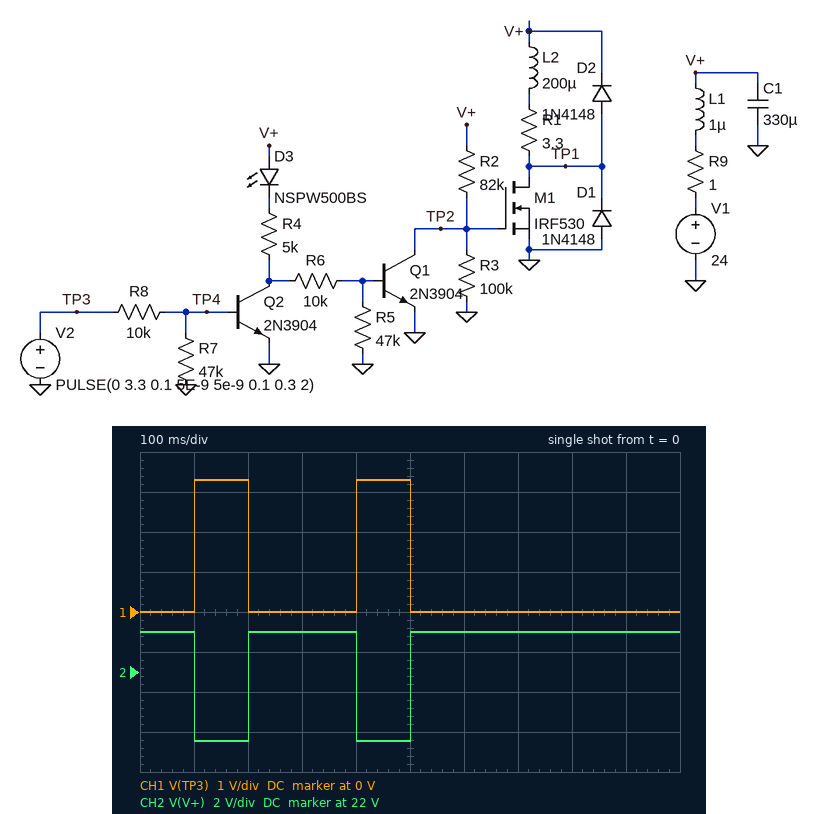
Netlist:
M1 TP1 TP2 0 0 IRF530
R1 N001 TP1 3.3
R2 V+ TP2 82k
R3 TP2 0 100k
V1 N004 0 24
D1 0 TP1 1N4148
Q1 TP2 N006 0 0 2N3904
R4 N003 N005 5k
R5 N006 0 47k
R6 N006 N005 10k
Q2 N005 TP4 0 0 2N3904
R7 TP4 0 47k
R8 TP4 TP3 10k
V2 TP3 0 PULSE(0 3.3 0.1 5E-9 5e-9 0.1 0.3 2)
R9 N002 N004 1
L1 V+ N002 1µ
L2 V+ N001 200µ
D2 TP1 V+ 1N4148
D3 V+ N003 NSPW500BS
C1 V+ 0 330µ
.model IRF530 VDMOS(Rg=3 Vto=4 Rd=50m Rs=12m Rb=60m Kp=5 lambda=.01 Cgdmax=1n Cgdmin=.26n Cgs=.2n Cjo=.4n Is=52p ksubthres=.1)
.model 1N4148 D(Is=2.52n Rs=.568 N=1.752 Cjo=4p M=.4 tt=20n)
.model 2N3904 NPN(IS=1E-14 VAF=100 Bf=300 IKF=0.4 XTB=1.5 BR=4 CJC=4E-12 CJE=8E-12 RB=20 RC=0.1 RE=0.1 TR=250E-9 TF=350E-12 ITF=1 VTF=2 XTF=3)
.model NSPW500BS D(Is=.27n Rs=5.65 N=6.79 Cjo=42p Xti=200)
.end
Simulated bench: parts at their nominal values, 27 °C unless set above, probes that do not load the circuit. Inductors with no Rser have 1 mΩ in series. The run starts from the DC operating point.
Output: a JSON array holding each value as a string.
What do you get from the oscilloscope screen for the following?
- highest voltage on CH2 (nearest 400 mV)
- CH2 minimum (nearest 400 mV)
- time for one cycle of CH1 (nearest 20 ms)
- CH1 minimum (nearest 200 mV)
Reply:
["24.0 V", "18.4 V", "300 ms", "0 V"]
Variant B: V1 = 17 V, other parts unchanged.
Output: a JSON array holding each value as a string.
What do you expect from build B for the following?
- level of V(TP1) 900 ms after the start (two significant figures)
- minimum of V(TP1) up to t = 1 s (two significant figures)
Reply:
["17 V", "490 mV"]
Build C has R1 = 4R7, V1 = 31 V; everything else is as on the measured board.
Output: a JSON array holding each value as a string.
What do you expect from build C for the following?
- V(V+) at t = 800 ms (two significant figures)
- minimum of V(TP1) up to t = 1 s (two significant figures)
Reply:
["31 V", "440 mV"]
